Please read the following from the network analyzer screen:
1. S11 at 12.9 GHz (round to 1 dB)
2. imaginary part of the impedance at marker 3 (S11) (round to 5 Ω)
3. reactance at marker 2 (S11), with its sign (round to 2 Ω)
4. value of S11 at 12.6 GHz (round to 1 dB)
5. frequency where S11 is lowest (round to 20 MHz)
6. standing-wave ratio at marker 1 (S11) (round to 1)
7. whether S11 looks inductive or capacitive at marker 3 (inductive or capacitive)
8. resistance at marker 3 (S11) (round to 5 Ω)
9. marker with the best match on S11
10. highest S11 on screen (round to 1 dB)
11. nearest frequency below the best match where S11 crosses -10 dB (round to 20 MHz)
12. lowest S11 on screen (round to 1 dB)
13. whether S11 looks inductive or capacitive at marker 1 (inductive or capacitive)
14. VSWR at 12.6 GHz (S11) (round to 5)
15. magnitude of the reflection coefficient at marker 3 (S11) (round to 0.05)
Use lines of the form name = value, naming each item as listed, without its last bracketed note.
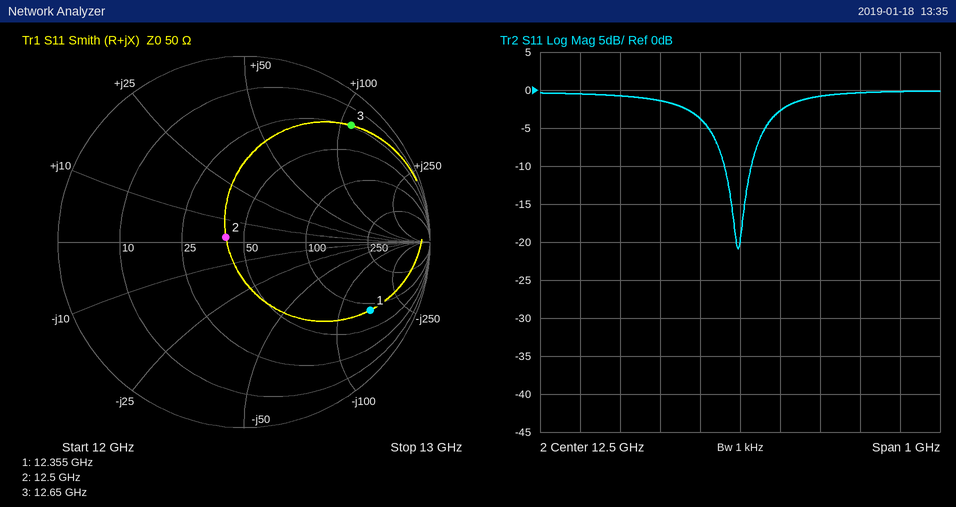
S11 at 12.9 GHz = 0 dB
imaginary part of the impedance at marker 3 (S11) = +110 Ω
reactance at marker 2 (S11), with its sign = +2 Ω
value of S11 at 12.6 GHz = -3 dB
frequency where S11 is lowest = 12.50 GHz
standing-wave ratio at marker 1 (S11) = 8
whether S11 looks inductive or capacitive at marker 3 = inductive
resistance at marker 3 (S11) = 25 Ω
marker with the best match on S11 = marker 2
highest S11 on screen = 0 dB
nearest frequency below the best match where S11 crosses -10 dB = 12.46 GHz
lowest S11 on screen = -21 dB
whether S11 looks inductive or capacitive at marker 1 = capacitive
VSWR at 12.6 GHz (S11) = 5
magnitude of the reflection coefficient at marker 3 (S11) = 0.85
